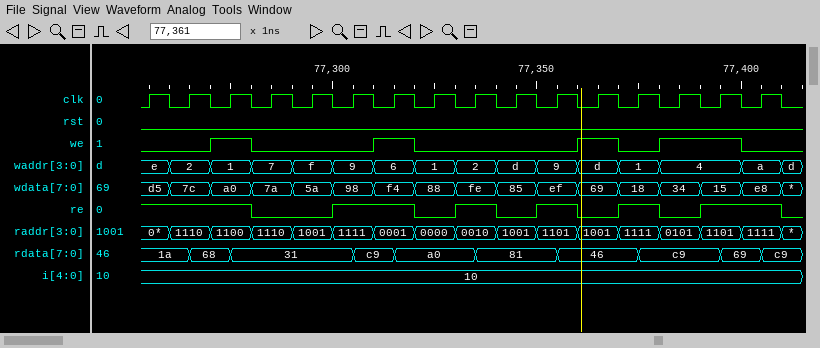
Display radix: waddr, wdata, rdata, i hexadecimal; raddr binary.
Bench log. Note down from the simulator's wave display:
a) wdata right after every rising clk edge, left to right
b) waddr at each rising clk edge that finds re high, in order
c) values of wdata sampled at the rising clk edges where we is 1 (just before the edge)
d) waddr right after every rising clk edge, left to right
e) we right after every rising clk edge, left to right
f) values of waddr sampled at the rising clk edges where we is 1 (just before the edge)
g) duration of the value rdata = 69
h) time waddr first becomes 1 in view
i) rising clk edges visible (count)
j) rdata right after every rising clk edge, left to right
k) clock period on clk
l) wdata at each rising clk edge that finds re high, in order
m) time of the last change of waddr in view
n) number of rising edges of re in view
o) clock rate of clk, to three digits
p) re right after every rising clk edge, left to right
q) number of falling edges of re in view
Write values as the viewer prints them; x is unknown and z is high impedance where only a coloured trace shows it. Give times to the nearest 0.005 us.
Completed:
d5, 7c, a0, 7a, 5a, 98, f4, 88, fe, 85, ef, 69, 18, 34, 15, e8
e, 2, 1, 9, 6, 2, 9, 1, 4, a
a0, f4, 69, 34, 15
e, 2, 1, 7, f, 9, 6, 1, 2, d, 9, d, 1, 4, 4, a
0 0 1 0 0 0 1 0 0 0 0 1 0 1 1 0
1, 6, d, 4, 4
0.01 us
77.27 us
16
1a, 68, 31, 31, 31, c9, a0, a0, 81, 81, 46, 46, c9, c9, 69, c9
0.01 us
d5, 7c, a0, 98, f4, fe, ef, 18, 15, e8
77.41 us
5
100 MHz
1 1 1 0 0 1 1 0 1 0 1 0 1 0 1 1
6
